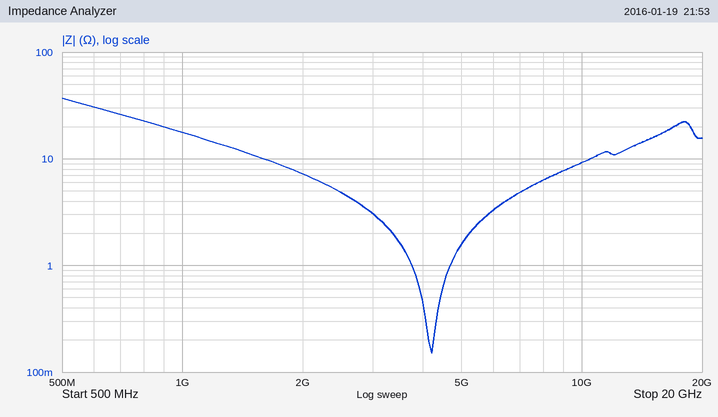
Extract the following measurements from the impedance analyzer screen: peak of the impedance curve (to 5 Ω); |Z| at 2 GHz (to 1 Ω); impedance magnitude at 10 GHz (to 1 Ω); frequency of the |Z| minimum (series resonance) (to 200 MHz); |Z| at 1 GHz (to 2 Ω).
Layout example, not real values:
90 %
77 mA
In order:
35 Ω
7 Ω
9 Ω
4.2 GHz
18 Ω
